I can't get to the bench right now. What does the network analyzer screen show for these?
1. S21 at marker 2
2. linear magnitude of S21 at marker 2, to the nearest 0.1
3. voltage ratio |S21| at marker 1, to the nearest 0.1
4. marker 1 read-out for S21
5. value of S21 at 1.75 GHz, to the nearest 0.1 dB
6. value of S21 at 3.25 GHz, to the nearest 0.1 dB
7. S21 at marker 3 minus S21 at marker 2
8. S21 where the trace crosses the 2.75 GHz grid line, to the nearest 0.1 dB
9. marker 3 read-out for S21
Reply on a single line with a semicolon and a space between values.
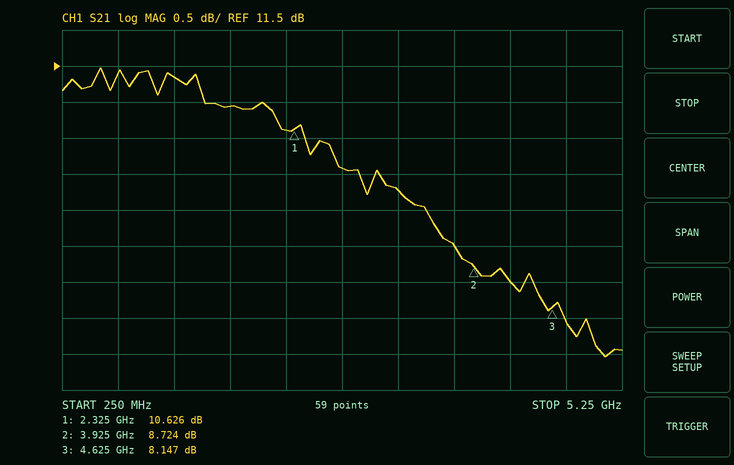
8.724 dB; 2.7; 3.4; 10.626 dB; 10.9 dB; 9.8 dB; -0.577 dB; 10.1 dB; 8.147 dB
